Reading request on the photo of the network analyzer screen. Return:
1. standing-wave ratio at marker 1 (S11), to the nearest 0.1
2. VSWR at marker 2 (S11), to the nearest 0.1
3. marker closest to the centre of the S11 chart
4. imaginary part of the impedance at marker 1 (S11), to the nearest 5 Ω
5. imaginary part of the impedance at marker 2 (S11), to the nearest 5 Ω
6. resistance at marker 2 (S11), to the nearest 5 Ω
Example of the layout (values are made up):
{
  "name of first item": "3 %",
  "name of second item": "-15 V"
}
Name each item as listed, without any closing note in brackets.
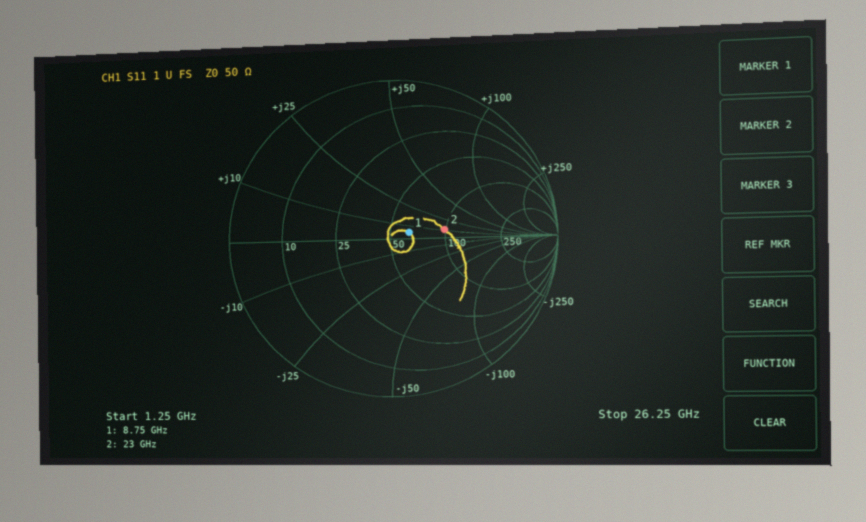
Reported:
{
  "standing-wave ratio at marker 1 (S11), to the nearest 0.1": "1.3",
  "VSWR at marker 2 (S11), to the nearest 0.1": "2.0",
  "marker closest to the centre of the S11 chart": "marker 1",
  "imaginary part of the impedance at marker 1 (S11), to the nearest 5 Ω": "+5 Ω",
  "imaginary part of the impedance at marker 2 (S11), to the nearest 5 Ω": "+10 Ω",
  "resistance at marker 2 (S11), to the nearest 5 Ω": "100 Ω"
}
